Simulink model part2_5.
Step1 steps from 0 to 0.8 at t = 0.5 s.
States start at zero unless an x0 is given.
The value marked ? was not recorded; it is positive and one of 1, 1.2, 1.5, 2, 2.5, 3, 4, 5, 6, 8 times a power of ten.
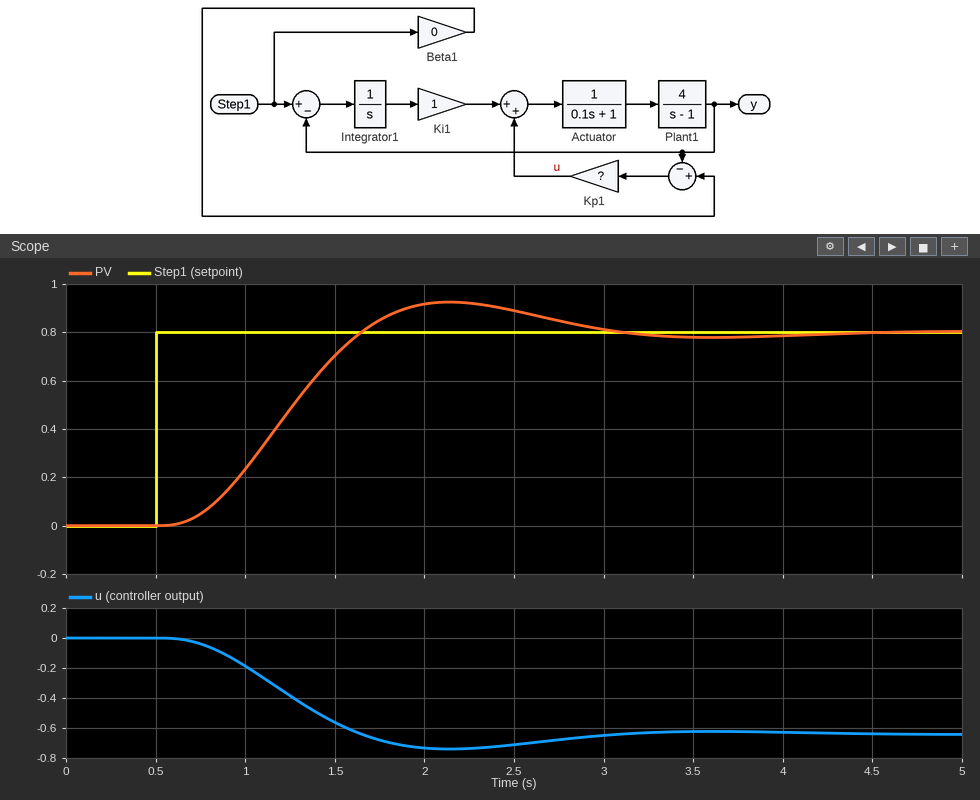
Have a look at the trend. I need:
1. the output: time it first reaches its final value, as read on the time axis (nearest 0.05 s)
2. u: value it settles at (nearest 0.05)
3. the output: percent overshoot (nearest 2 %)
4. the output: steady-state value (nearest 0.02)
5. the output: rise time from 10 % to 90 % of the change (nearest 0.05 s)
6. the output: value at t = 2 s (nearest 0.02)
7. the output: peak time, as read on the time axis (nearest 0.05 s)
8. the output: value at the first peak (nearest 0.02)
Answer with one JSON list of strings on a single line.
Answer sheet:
["1.65 s", "-0.65", "16 %", "0.80", "0.70 s", "0.92", "2.15 s", "0.92"]
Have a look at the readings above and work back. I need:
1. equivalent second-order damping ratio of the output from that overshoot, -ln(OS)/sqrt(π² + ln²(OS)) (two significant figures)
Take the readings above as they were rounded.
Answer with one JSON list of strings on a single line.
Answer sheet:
["0.50"]
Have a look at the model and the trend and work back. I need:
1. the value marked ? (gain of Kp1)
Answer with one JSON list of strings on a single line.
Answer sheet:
["0.8"]
